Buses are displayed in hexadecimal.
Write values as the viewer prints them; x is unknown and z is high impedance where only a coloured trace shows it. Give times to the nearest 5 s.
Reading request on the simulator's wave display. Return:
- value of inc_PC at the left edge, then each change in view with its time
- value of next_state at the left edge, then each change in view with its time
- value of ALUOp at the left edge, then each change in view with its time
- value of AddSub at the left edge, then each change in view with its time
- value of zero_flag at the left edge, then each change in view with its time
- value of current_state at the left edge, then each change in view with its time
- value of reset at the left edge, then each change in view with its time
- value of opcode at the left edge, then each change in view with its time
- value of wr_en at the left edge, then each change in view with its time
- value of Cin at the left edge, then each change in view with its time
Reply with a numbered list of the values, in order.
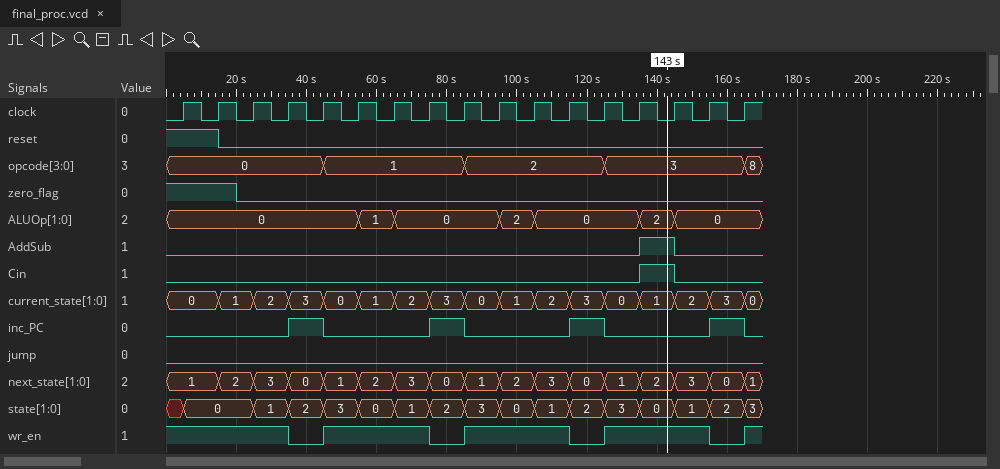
1. 0, 1 at 35 s, 0 at 45 s, 1 at 75 s, 0 at 85 s, 1 at 115 s, 0 at 125 s, 1 at 155 s, 0 at 165 s
2. 1, 2 at 15 s, 3 at 25 s, 0 at 35 s, 1 at 45 s, 2 at 55 s, 3 at 65 s, 0 at 75 s, 1 at 85 s, 2 at 95 s, 3 at 105 s, 0 at 115 s, 1 at 125 s, 2 at 135 s, 3 at 145 s, 0 at 155 s, 1 at 165 s
3. 0, 1 at 55 s, 0 at 65 s, 2 at 95 s, 0 at 105 s, 2 at 135 s, 0 at 145 s
4. 0, 1 at 135 s, 0 at 145 s
5. 1, 0 at 20 s
6. 0, 1 at 15 s, 2 at 25 s, 3 at 35 s, 0 at 45 s, 1 at 55 s, 2 at 65 s, 3 at 75 s, 0 at 85 s, 1 at 95 s, 2 at 105 s, 3 at 115 s, 0 at 125 s, 1 at 135 s, 2 at 145 s, 3 at 155 s, 0 at 165 s
7. 1, 0 at 15 s
8. 0, 1 at 45 s, 2 at 85 s, 3 at 125 s, 8 at 165 s
9. 1, 0 at 35 s, 1 at 45 s, 0 at 75 s, 1 at 85 s, 0 at 115 s, 1 at 125 s, 0 at 155 s, 1 at 165 s
10. 0, 1 at 135 s, 0 at 145 s
